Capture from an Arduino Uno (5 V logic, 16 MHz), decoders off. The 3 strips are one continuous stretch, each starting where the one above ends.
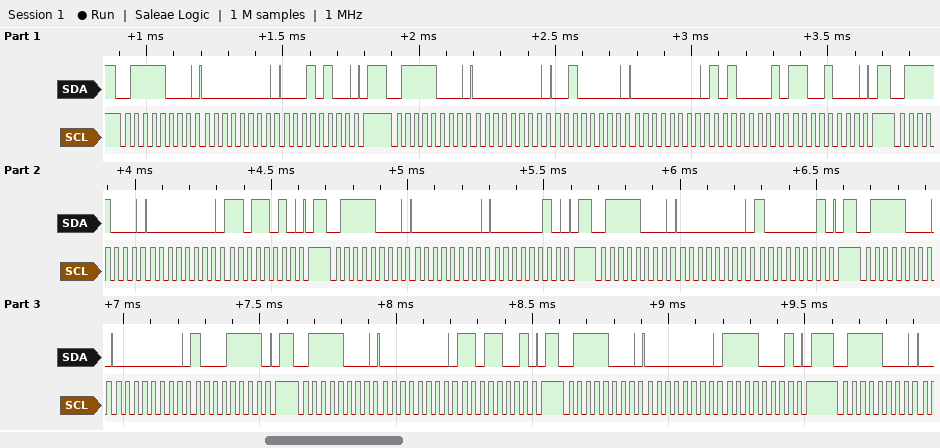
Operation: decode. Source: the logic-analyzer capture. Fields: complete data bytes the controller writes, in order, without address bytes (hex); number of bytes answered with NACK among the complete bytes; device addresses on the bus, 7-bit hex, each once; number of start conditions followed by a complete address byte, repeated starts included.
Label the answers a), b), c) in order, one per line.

a) 00 14 00 20 00 A1 C8 00 DA 00 02 00 81 00 8F 00 D9 00 F1
b) 0
c) 0x3C
d) 9
